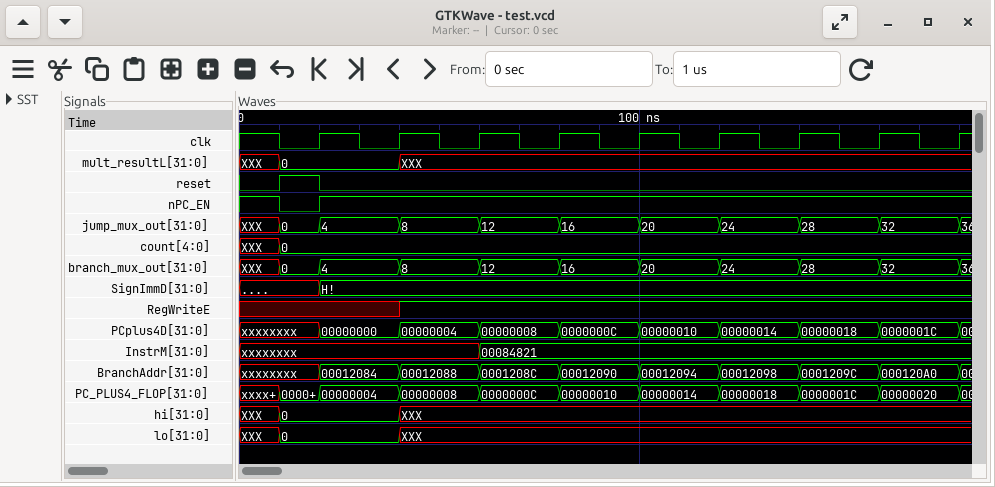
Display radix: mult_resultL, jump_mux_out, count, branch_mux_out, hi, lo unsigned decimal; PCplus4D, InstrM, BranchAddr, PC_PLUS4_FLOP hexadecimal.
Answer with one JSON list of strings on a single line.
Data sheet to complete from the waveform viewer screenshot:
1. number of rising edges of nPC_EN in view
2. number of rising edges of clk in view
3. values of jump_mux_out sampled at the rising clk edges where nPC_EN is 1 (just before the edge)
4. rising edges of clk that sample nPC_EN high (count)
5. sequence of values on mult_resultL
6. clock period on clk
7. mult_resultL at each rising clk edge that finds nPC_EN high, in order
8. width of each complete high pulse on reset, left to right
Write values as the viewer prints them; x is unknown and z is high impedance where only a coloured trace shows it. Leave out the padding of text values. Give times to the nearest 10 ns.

["1", "9", "4, 8, 12, 16, 20, 24, 28, 32", "8", "XXX, 0, XXX", "20 ns", "0, XXX, XXX, XXX, XXX, XXX, XXX, XXX", "10 ns"]
